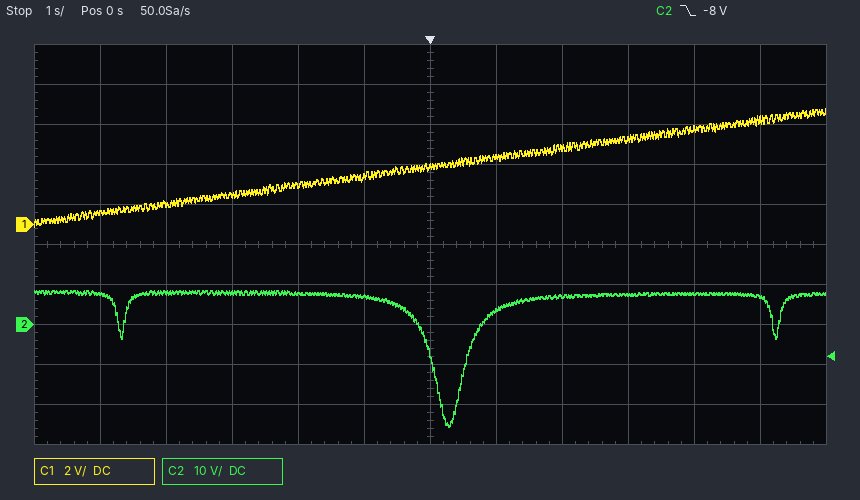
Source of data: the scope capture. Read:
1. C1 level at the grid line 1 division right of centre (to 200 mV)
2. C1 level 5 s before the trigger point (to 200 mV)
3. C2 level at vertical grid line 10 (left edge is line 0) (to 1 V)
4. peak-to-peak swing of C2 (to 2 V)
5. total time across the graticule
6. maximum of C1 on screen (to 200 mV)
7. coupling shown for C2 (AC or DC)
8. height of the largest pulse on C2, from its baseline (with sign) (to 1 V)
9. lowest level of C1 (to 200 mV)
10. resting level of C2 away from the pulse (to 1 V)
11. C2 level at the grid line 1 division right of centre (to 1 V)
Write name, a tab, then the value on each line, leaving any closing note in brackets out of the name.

C1 level at the grid line 1 division right of centre	3.4 V
C1 level 5 s before the trigger point	600 mV
C2 level at vertical grid line 10 (left edge is line 0)	8 V
peak-to-peak swing of C2	34 V
total time across the graticule	12 s
maximum of C1 on screen	5.8 V
coupling shown for C2	DC
height of the largest pulse on C2, from its baseline (with sign)	-33 V
lowest level of C1	0.0 V
resting level of C2 away from the pulse	8 V
C2 level at the grid line 1 division right of centre	4 V
